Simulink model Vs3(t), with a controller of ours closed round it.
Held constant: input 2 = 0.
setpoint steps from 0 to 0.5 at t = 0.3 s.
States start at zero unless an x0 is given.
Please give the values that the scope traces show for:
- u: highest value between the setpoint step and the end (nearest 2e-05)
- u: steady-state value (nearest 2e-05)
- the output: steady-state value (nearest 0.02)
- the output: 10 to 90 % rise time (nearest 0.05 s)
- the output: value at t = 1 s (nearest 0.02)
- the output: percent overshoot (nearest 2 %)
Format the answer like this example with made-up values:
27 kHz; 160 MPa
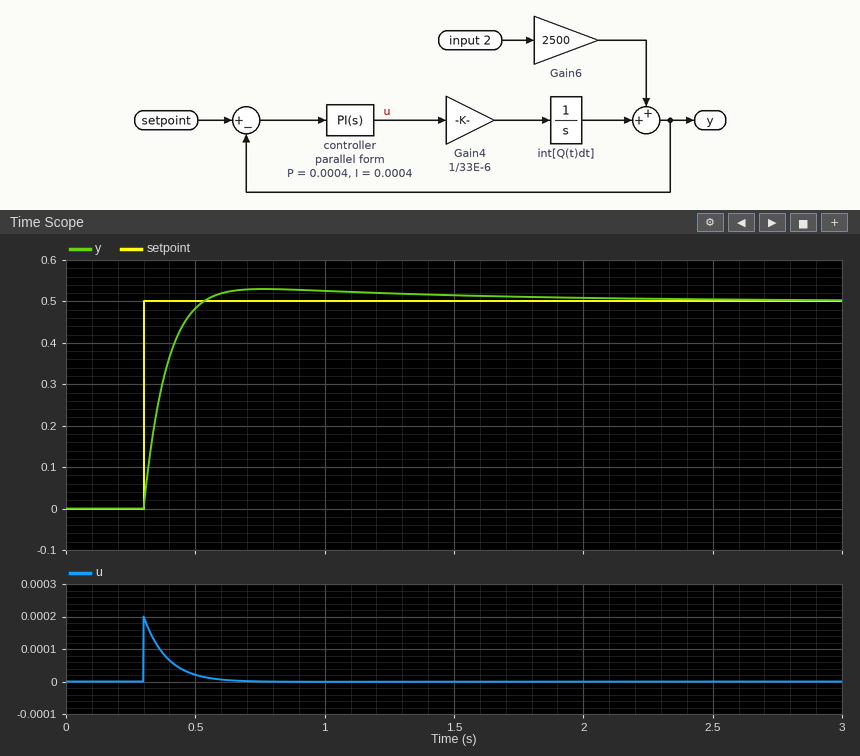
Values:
0.00020; 0.00000; 0.50; 0.15 s; 0.52; 6 %
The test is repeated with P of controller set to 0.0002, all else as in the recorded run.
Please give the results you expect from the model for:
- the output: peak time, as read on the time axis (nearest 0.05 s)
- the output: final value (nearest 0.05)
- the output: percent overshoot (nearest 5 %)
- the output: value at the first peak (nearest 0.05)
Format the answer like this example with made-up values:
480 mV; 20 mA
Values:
0.90 s; 0.50; 15 %; 0.60
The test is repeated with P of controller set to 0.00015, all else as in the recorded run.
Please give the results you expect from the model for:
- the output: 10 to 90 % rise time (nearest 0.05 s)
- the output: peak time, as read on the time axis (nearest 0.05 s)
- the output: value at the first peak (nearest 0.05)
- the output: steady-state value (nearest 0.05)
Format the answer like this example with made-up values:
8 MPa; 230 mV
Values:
0.25 s; 0.95 s; 0.60; 0.50
